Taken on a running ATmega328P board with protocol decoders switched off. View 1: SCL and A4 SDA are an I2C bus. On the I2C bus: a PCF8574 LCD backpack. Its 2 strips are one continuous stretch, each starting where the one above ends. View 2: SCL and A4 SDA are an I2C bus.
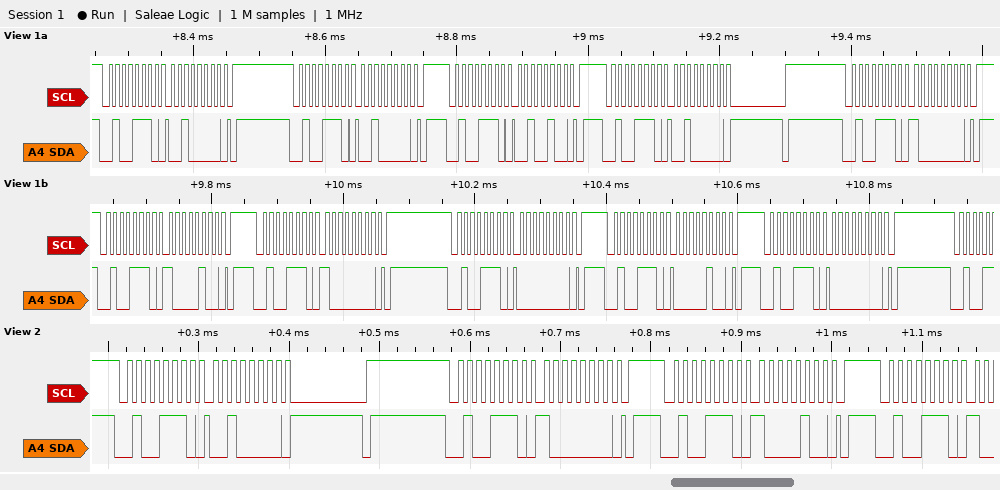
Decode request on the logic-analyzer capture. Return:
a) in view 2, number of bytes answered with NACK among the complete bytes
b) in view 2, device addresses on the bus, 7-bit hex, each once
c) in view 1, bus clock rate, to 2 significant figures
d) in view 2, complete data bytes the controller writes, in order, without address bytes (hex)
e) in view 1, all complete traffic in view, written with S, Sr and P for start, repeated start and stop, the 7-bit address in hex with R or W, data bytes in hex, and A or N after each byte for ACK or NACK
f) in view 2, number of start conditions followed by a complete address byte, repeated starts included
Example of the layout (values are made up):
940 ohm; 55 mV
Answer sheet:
0; 0x27; 100 kHz; 20 80 84; S 27W A 20 A P S 27W A 20 A P S 27W A 24 A P S 27W A 20 A P S 27W A 80 A P S 27W A 84 A P S 27W A 80 A P S 27W A 00 A P S 27W A 04 A P S 27W A 00 A P; 4
